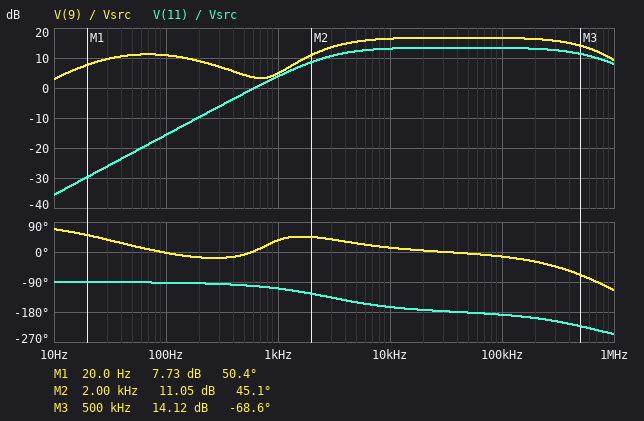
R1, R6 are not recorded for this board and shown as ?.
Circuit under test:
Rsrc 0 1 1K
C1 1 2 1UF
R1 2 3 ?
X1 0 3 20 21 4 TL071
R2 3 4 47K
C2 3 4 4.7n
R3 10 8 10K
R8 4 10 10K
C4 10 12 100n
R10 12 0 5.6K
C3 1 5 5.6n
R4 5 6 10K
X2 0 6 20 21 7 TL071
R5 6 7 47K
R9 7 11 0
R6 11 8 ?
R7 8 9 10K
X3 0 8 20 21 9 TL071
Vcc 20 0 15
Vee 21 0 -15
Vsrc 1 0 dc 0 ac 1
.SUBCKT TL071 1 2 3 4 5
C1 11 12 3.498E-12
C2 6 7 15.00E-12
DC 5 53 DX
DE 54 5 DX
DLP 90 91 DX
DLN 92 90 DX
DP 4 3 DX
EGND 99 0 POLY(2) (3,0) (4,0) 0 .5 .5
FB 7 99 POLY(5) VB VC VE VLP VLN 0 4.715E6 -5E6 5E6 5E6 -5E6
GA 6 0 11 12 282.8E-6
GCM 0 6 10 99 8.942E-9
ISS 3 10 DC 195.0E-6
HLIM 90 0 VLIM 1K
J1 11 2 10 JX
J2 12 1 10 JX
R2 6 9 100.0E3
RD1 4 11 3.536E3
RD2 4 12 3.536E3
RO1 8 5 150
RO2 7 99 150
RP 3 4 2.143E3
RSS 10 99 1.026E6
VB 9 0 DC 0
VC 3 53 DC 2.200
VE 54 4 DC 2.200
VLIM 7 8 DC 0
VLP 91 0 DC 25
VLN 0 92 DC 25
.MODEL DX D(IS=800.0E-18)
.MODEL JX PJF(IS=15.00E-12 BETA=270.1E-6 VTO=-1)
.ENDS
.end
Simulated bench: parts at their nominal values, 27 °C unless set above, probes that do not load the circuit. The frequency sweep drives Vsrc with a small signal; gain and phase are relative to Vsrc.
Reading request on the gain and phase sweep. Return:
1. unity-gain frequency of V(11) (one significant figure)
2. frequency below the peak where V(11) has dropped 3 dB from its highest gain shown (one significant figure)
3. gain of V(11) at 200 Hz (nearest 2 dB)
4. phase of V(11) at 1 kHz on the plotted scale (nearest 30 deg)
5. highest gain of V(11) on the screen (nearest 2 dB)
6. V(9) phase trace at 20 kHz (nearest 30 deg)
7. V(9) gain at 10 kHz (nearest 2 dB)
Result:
600 Hz
3 kHz
-10 dB
-120 deg
14 dB
0 deg
16 dB
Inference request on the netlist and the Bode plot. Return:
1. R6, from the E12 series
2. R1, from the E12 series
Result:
6.8 kΩ
5.6 kΩ
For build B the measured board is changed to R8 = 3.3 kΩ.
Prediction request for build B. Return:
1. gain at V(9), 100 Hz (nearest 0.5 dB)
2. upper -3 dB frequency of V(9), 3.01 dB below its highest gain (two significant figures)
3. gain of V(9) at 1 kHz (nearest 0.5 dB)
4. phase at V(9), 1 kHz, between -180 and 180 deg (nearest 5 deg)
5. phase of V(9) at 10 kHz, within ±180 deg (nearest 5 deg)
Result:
15.0 dB
530 kHz
6.5 dB
0 deg
10 deg
